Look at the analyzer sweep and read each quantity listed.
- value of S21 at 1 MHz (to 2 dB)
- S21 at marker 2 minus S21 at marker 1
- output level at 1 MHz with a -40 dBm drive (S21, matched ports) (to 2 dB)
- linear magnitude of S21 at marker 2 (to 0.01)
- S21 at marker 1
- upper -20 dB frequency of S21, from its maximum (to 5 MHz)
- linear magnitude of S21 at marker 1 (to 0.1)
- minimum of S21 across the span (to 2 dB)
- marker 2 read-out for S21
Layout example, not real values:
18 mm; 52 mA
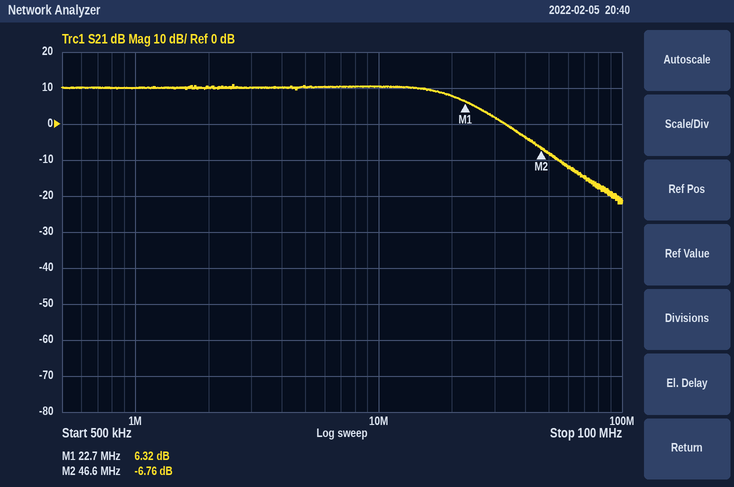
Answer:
10 dB; -13.08 dB; -30 dBm; 0.46; 6.32 dB; 50 MHz; 2.1; -22 dB; -6.76 dB
